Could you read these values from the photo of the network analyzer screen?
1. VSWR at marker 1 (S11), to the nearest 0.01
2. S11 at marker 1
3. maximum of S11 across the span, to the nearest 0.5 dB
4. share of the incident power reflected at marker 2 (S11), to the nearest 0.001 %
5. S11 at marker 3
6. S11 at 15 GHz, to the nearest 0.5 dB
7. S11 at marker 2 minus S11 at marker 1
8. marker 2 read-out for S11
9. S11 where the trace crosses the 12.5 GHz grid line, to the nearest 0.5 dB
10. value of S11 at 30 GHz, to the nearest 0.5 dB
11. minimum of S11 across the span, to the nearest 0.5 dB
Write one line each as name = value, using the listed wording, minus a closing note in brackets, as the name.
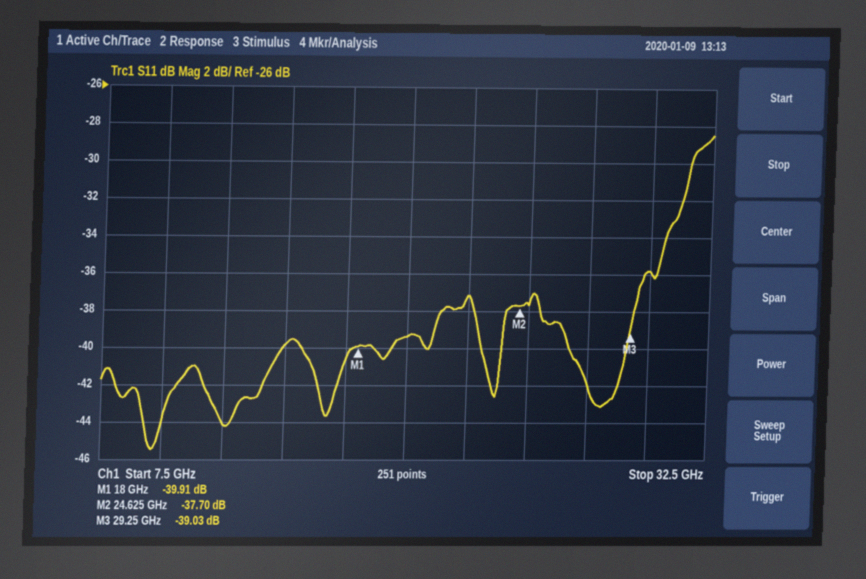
VSWR at marker 1 (S11), to the nearest 0.01 = 1.02
S11 at marker 1 = -39.91 dB
maximum of S11 across the span, to the nearest 0.5 dB = -28.5 dB
share of the incident power reflected at marker 2 (S11), to the nearest 0.001 % = 0.017 %
S11 at marker 3 = -39.03 dB
S11 at 15 GHz, to the nearest 0.5 dB = -40.0 dB
S11 at marker 2 minus S11 at marker 1 = 2.21 dB
marker 2 read-out for S11 = -37.70 dB
S11 where the trace crosses the 12.5 GHz grid line, to the nearest 0.5 dB = -44.0 dB
value of S11 at 30 GHz, to the nearest 0.5 dB = -36.0 dB
minimum of S11 across the span, to the nearest 0.5 dB = -45.5 dB
